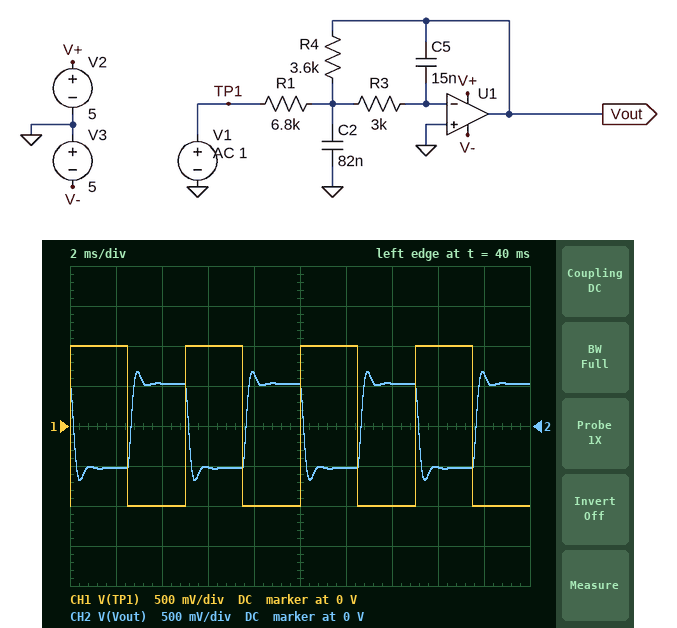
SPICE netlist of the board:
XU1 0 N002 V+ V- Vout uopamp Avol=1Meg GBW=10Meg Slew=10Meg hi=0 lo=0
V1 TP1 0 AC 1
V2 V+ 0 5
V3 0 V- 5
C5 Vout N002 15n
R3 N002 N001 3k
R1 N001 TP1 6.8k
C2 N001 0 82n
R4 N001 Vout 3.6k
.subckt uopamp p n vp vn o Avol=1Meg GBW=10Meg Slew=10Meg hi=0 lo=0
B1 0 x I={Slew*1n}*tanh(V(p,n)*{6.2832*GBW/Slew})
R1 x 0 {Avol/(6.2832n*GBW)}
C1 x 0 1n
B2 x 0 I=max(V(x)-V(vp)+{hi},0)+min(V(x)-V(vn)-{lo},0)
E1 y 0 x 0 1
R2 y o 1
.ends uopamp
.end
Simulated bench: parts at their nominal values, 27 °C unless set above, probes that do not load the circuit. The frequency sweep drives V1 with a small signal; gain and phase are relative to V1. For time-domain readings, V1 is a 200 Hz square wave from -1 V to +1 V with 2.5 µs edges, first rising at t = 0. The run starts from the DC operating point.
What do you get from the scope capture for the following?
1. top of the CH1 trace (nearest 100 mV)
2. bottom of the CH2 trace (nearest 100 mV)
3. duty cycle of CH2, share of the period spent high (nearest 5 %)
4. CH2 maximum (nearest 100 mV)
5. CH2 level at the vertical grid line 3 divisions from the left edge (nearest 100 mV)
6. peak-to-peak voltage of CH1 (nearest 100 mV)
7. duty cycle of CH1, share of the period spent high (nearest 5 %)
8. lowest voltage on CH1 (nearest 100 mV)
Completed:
1.0 V
-700 mV
50 %
700 mV
-500 mV
2.0 V
50 %
-1.0 V
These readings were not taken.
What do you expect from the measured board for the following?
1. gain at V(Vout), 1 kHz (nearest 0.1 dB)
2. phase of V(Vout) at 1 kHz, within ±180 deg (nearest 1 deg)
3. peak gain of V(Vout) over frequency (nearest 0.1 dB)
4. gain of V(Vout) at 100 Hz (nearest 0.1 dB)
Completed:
-4.7 dB
122 deg
-4.6 dB
-5.5 dB
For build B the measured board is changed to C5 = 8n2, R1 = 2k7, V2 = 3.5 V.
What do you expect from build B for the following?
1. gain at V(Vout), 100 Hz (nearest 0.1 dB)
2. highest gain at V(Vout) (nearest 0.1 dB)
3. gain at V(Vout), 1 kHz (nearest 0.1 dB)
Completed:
2.5 dB
3.6 dB
3.4 dB
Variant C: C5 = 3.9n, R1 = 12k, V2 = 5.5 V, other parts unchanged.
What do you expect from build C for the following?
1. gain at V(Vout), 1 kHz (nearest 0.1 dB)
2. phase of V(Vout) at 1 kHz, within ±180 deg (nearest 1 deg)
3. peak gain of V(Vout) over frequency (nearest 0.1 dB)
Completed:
-9.4 dB
168 deg
-4.1 dB
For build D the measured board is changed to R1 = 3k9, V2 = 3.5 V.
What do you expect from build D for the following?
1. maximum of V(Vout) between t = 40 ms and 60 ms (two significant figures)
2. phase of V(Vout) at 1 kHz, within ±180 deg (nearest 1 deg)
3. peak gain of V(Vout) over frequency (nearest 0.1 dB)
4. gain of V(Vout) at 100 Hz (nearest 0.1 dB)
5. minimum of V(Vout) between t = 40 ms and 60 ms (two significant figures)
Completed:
1.1 V
118 deg
-0.4 dB
-0.7 dB
-1.1 V
